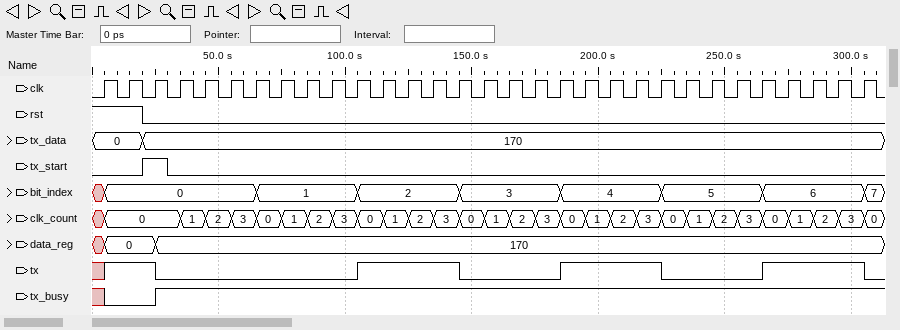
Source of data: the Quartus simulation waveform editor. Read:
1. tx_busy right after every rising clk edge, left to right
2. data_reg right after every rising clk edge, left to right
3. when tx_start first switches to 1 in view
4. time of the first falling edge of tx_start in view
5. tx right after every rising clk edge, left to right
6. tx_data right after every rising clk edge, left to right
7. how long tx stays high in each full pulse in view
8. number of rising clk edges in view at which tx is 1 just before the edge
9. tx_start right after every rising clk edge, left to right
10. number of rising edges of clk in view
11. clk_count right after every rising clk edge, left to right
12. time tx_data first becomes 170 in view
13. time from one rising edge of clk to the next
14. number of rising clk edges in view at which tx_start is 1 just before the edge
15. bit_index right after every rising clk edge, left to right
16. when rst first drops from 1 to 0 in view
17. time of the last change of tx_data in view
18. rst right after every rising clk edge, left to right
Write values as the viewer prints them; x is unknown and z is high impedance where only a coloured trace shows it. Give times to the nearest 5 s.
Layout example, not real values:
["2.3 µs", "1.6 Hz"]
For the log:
["0 0 1 1 1 1 1 1 1 1 1 1 1 1 1 1 1 1 1 1 1 1 1 1 1 1 1 1 1 1 1", "0, 0, 170, 170, 170, 170, 170, 170, 170, 170, 170, 170, 170, 170, 170, 170, 170, 170, 170, 170, 170, 170, 170, 170, 170, 170, 170, 170, 170, 170, 170", "20 s", "30 s", "1 1 0 0 0 0 0 0 0 0 1 1 1 1 0 0 0 0 1 1 1 1 0 0 0 0 1 1 1 1 0", "0, 0, 170, 170, 170, 170, 170, 170, 170, 170, 170, 170, 170, 170, 170, 170, 170, 170, 170, 170, 170, 170, 170, 170, 170, 170, 170, 170, 170, 170, 170", "40 s, 40 s, 40 s", "14", "0 0 1 0 0 0 0 0 0 0 0 0 0 0 0 0 0 0 0 0 0 0 0 0 0 0 0 0 0 0 0", "31", "0, 0, 0, 1, 2, 3, 0, 1, 2, 3, 0, 1, 2, 3, 0, 1, 2, 3, 0, 1, 2, 3, 0, 1, 2, 3, 0, 1, 2, 3, 0", "20 s", "10 s", "1", "0, 0, 0, 0, 0, 0, 1, 1, 1, 1, 2, 2, 2, 2, 3, 3, 3, 3, 4, 4, 4, 4, 5, 5, 5, 5, 6, 6, 6, 6, 7", "20 s", "20 s", "1 1 0 0 0 0 0 0 0 0 0 0 0 0 0 0 0 0 0 0 0 0 0 0 0 0 0 0 0 0 0"]
